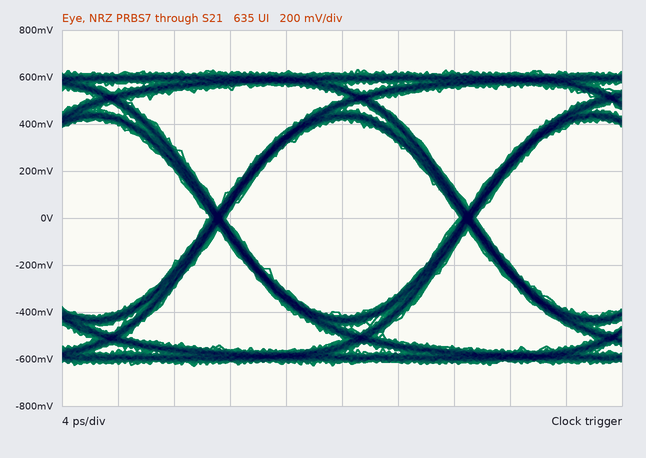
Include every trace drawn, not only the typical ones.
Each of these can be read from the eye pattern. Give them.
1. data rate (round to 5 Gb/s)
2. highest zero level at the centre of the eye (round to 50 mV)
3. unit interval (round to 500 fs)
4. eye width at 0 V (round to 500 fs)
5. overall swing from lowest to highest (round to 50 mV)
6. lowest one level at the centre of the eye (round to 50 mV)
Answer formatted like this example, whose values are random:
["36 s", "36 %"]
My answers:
["55 Gb/s", "-400 mV", "18.0 ps", "16.5 ps", "1.25 V", "400 mV"]
